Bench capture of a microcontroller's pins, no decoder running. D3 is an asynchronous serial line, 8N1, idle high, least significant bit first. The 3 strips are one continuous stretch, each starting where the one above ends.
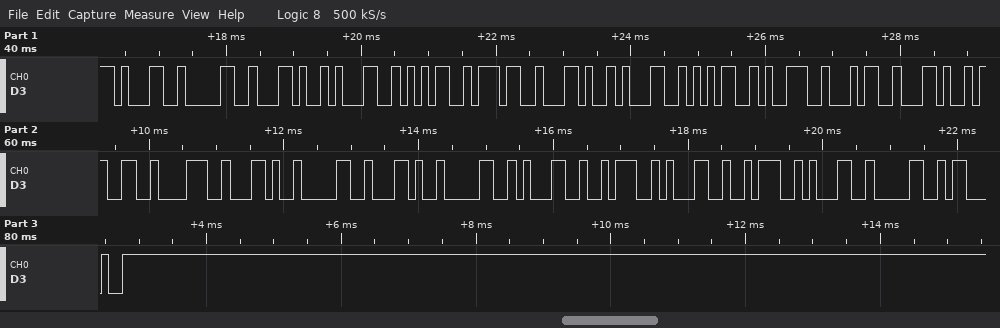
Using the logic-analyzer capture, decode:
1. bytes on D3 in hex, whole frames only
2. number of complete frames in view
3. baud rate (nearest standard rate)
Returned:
31 30 2C 31 35 37 2C 31 35 39 34 2C 33 38 2C 30 2C 30 31 3A 31 3A 31 30 23
25
9600 baud
